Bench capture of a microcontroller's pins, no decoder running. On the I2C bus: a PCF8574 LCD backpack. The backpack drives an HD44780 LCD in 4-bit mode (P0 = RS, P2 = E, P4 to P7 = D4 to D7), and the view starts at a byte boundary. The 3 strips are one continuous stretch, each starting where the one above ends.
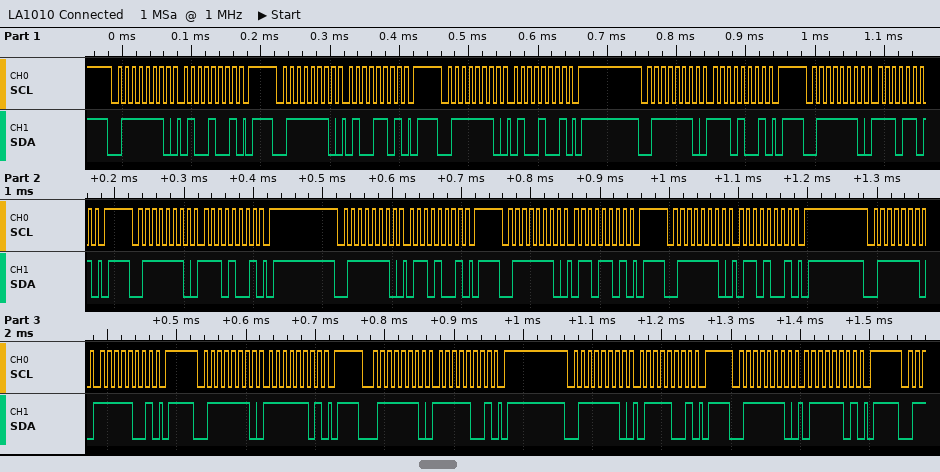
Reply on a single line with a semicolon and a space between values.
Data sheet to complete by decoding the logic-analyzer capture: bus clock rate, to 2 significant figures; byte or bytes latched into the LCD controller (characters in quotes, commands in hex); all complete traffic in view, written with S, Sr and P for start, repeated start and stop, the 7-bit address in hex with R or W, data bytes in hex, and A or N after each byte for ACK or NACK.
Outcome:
100 kHz; 'N' 'o'; S 3FW A 49 A P S 3FW A 4D A P S 3FW A 49 A P S 3FW A E9 A P S 3FW A ED A P S 3FW A E9 A P S 3FW A 69 A P S 3FW A 6D A P S 3FW A 69 A P S 3FW A F9 A P S 3FW A FD A P S 3FW A F9 A P S 3FW A 79 A P S 3FW A 7D A P
